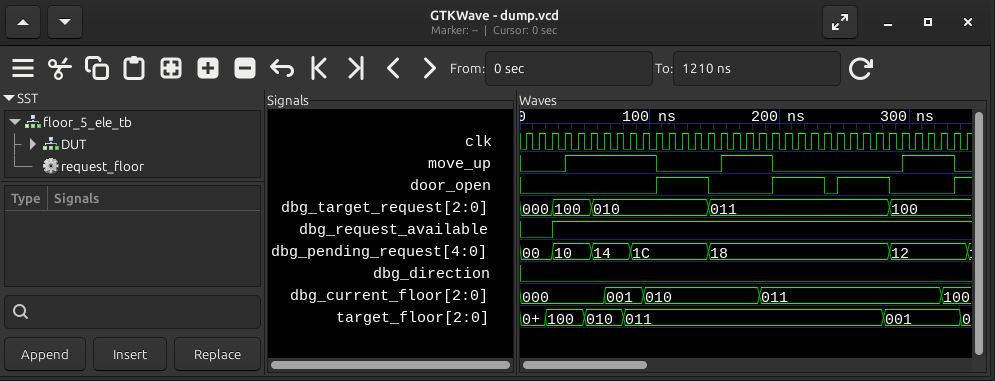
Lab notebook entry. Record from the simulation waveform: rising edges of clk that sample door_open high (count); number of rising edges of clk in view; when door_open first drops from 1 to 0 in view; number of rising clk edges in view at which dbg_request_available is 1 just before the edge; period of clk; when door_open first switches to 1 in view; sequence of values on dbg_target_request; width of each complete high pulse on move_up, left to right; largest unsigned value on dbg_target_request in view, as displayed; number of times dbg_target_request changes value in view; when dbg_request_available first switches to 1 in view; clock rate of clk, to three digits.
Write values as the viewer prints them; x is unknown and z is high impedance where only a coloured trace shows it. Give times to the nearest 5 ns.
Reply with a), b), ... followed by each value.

a) 13
b) 35
c) 145 ns
d) 32
e) 10 ns
f) 105 ns
g) 000, 100, 010, 011, 100
h) 70 ns, 40 ns, 40 ns
i) 100
j) 4
k) 25 ns
l) 100 MHz
